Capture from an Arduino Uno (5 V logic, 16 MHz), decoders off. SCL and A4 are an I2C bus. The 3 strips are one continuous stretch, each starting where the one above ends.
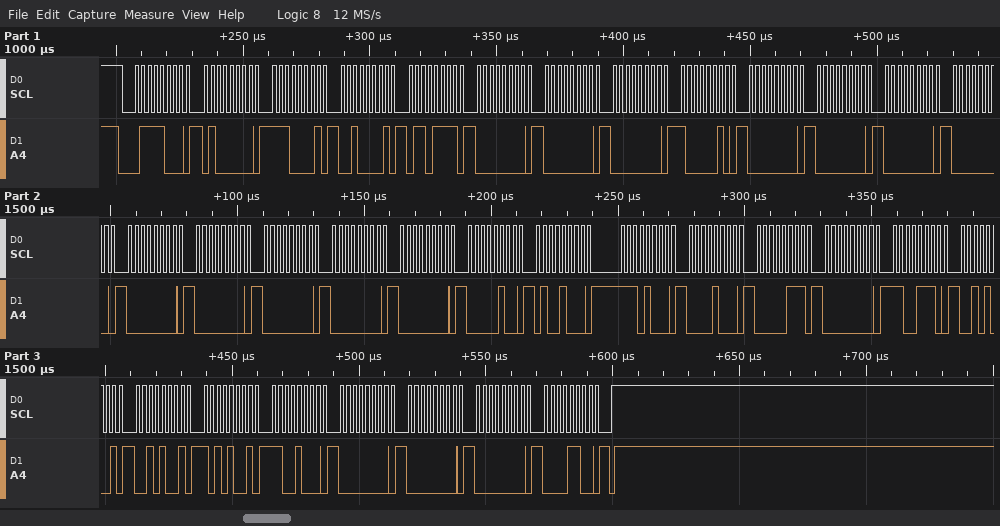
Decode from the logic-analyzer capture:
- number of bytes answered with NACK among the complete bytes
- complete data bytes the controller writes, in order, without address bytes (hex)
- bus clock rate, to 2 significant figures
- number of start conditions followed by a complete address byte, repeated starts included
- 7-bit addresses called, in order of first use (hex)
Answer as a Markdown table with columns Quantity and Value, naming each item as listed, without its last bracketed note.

| Quantity | Value |
|---|---|
| number of bytes answered with NACK among the complete bytes | 0 |
| complete data bytes the controller writes, in order, without address bytes | 40 E1 21 6F 00 00 00 82 00 00 00 00 00 00 00 00 00 04 48 E8 08 07 00 CE 29 29 A9 C8 00 00 00 0C |
| bus clock rate, to 2 significant figures | 400 kHz |
| number of start conditions followed by a complete address byte, repeated starts included | 1 |
| 7-bit addresses called, in order of first use | 0x3C |
